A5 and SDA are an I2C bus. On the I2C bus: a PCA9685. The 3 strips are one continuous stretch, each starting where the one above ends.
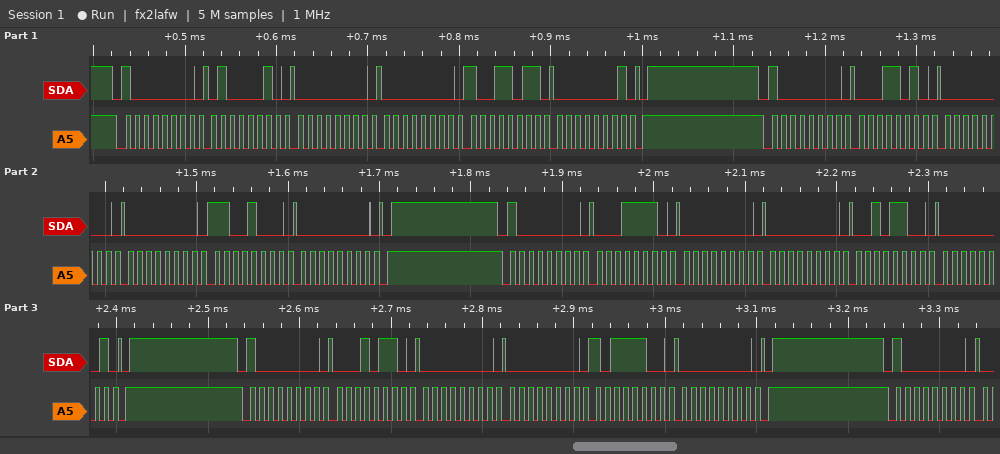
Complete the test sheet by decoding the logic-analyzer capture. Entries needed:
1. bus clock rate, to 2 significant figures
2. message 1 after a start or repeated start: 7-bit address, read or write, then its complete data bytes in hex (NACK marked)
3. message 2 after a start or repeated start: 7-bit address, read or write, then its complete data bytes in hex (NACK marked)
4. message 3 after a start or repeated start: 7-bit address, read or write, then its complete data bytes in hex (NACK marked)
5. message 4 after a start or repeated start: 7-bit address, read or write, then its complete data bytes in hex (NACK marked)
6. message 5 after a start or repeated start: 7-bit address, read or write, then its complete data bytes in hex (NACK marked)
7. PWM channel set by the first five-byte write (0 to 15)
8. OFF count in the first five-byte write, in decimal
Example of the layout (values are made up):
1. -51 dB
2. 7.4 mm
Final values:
1. 100 kHz
2. 0x40 write: 42 00 00 9B 01
3. 0x40 write: 1A 00 00 C8 00
4. 0x40 write: 1E 00 00 2C 01
5. 0x40 write: 16 00 00 BC 00
6. 0x40 write
7. 15
8. 411
